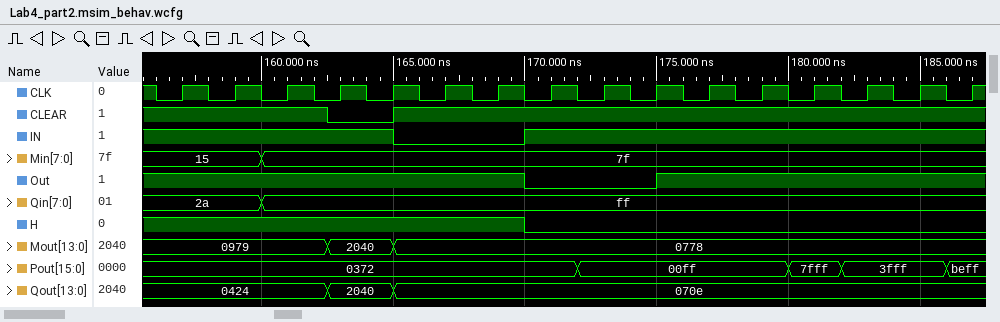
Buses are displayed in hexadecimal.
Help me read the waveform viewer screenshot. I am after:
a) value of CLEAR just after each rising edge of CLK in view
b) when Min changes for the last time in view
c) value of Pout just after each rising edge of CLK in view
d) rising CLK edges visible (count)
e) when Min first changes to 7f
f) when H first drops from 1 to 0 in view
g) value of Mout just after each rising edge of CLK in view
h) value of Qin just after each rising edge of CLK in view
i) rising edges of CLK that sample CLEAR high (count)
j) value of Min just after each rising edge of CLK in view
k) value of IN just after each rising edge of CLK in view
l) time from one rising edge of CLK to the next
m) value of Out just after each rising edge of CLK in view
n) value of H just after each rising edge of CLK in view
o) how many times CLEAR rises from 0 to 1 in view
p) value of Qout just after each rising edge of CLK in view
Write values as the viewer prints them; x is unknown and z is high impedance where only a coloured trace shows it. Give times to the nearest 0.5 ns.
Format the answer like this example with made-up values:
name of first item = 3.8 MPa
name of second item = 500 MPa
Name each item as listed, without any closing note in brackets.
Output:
value of CLEAR just after each rising edge of CLK in view = 1 1 1 0 1 1 1 1 1 1 1 1 1 1 1 1
when Min changes for the last time in view = 160 ns
value of Pout just after each rising edge of CLK in view = 0372, 0372, 0372, 0372, 0372, 0372, 0372, 0372, 00ff, 00ff, 00ff, 00ff, 7fff, 3fff, 3fff, beff
rising CLK edges visible = 16
when Min first changes to 7f = 160 ns
when H first drops from 1 to 0 in view = 170 ns
value of Mout just after each rising edge of CLK in view = 0979, 0979, 0979, 2040, 0778, 0778, 0778, 0778, 0778, 0778, 0778, 0778, 0778, 0778, 0778, 0778
value of Qin just after each rising edge of CLK in view = 2a, 2a, ff, ff, ff, ff, ff, ff, ff, ff, ff, ff, ff, ff, ff, ff
rising edges of CLK that sample CLEAR high = 14
value of Min just after each rising edge of CLK in view = 15, 15, 7f, 7f, 7f, 7f, 7f, 7f, 7f, 7f, 7f, 7f, 7f, 7f, 7f, 7f
value of IN just after each rising edge of CLK in view = 1 1 1 1 0 0 0 1 1 1 1 1 1 1 1 1
time from one rising edge of CLK to the next = 2 ns
value of Out just after each rising edge of CLK in view = 1 1 1 1 1 1 1 0 0 1 1 1 1 1 1 1
value of H just after each rising edge of CLK in view = 1 1 1 1 1 1 1 0 0 0 0 0 0 0 0 0
how many times CLEAR rises from 0 to 1 in view = 1
value of Qout just after each rising edge of CLK in view = 0424, 0424, 0424, 2040, 070e, 070e, 070e, 070e, 070e, 070e, 070e, 070e, 070e, 070e, 070e, 070e
